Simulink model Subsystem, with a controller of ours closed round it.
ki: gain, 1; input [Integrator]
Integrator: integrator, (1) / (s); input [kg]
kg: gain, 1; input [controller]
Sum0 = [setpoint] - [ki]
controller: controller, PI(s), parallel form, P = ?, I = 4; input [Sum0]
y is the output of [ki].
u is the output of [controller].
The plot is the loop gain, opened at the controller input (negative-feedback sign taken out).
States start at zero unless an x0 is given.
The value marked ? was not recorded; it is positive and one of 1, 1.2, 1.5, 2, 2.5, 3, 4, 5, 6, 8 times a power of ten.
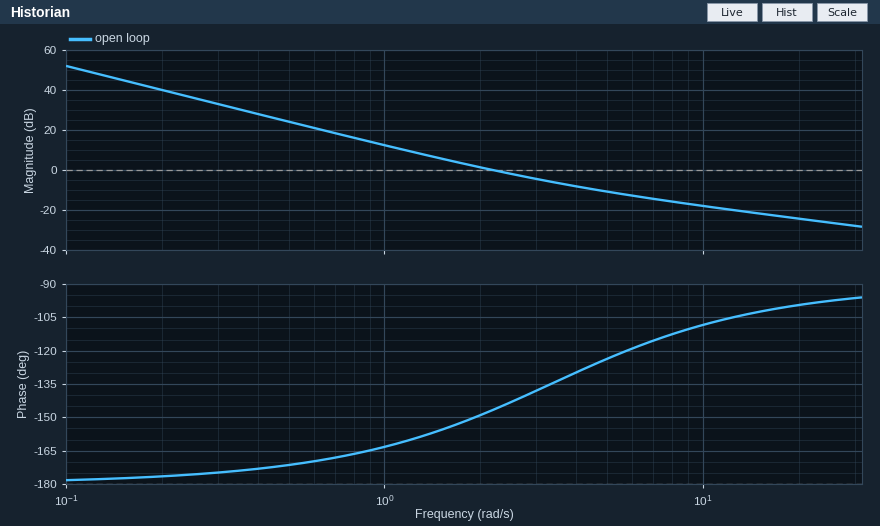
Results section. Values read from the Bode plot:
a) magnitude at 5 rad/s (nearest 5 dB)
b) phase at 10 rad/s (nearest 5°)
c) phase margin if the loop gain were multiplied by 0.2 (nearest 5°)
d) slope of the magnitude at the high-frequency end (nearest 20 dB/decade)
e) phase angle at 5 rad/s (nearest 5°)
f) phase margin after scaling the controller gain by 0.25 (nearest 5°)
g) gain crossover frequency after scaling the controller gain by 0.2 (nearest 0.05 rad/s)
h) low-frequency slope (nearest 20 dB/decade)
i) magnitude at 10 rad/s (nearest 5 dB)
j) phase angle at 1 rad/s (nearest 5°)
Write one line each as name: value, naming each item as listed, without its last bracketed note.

magnitude at 5 rad/s: -10 dB
phase at 10 rad/s: -110°
phase margin if the loop gain were multiplied by 0.2: 15°
slope of the magnitude at the high-frequency end: -20 dB/decade
phase angle at 5 rad/s: -125°
phase margin after scaling the controller gain by 0.25: 15°
gain crossover frequency after scaling the controller gain by 0.2: 0.90 rad/s
low-frequency slope: -40 dB/decade
magnitude at 10 rad/s: -20 dB
phase angle at 1 rad/s: -165°
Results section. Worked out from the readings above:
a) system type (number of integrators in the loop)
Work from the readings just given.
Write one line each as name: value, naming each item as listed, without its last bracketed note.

system type: 2
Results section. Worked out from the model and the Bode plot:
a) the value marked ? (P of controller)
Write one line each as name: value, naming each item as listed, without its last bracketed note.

the value marked ?: 1.2
